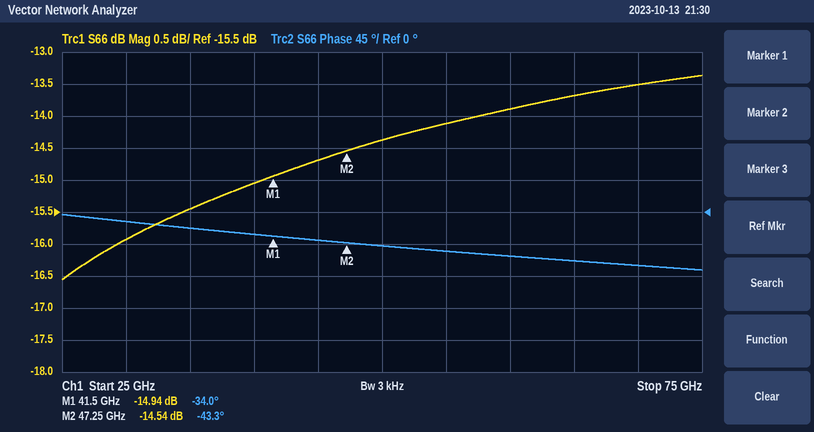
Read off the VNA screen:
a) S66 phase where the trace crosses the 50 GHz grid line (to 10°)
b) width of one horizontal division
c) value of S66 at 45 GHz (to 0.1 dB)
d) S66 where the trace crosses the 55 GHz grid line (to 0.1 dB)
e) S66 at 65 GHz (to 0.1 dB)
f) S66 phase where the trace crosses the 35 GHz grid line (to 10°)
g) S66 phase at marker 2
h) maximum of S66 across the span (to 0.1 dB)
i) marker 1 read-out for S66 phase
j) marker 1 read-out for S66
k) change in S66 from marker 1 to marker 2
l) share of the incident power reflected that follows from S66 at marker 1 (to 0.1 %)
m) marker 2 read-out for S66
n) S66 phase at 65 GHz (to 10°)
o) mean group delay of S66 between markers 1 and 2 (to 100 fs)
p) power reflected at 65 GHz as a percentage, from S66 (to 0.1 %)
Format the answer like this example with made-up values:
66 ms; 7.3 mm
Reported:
-50°; 5 GHz; -14.7 dB; -14.1 dB; -13.7 dB; -20°; -43.3°; -13.4 dB; -34.0°; -14.94 dB; 0.40 dB; 3.2 %; -14.54 dB; -70°; 4.5 ps; 4.3 %
